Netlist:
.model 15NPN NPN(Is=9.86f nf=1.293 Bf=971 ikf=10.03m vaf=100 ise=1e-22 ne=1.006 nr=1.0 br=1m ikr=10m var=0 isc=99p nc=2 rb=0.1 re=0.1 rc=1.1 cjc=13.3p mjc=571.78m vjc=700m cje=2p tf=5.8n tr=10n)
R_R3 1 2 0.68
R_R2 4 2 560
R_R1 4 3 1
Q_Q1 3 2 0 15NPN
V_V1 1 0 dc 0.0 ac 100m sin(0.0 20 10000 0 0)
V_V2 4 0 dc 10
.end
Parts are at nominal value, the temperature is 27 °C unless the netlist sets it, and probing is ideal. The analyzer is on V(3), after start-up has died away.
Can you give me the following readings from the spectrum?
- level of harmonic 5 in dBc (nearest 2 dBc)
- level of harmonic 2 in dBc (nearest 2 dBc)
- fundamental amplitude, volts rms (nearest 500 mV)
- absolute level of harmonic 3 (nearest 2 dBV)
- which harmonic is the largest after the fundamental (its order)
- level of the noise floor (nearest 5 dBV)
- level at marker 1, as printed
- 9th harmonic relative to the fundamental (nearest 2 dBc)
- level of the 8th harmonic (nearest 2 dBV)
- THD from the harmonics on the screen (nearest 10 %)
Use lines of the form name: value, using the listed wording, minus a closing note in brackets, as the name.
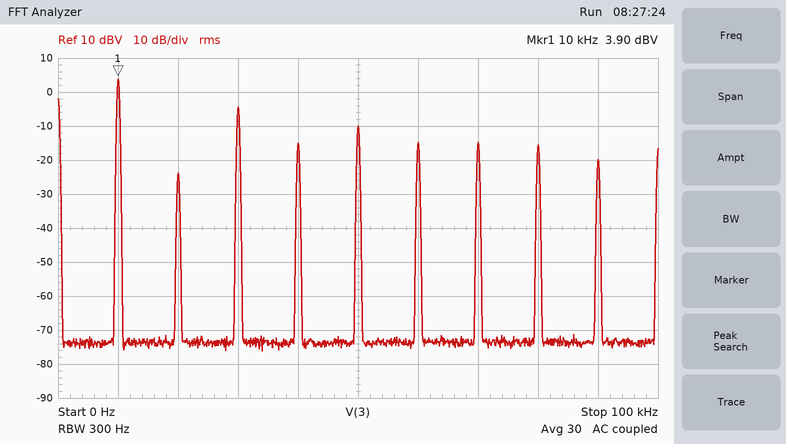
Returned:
level of harmonic 5 in dBc: -14 dBc
level of harmonic 2 in dBc: -28 dBc
fundamental amplitude, volts rms: 1.5 V
absolute level of harmonic 3: -4 dBV
which harmonic is the largest after the fundamental: 3
level of the noise floor: -75 dBV
level at marker 1, as printed: 3.90 dBV
9th harmonic relative to the fundamental: -24 dBc
level of the 8th harmonic: -16 dBV
THD from the harmonics on the screen: 50 %
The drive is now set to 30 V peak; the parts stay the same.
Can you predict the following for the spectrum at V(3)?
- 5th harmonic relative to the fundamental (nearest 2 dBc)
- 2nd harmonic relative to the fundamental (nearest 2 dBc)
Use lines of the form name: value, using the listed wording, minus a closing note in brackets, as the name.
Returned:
5th harmonic relative to the fundamental: -12 dBc
2nd harmonic relative to the fundamental: -24 dBc
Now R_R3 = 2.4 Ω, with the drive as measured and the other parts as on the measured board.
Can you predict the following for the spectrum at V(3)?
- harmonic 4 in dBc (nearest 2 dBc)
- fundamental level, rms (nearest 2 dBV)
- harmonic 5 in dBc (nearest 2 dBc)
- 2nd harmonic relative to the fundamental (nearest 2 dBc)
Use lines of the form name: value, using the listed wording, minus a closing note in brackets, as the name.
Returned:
harmonic 4 in dBc: -16 dBc
fundamental level, rms: 4 dBV
harmonic 5 in dBc: -20 dBc
2nd harmonic relative to the fundamental: -16 dBc
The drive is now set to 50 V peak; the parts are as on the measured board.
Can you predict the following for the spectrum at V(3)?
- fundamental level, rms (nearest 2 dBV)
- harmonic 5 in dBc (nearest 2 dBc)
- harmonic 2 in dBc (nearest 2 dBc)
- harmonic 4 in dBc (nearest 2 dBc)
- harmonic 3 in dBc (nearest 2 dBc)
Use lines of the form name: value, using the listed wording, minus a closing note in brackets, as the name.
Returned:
fundamental level, rms: 0 dBV
harmonic 5 in dBc: -8 dBc
harmonic 2 in dBc: -10 dBc
harmonic 4 in dBc: -40 dBc
harmonic 3 in dBc: -4 dBc
